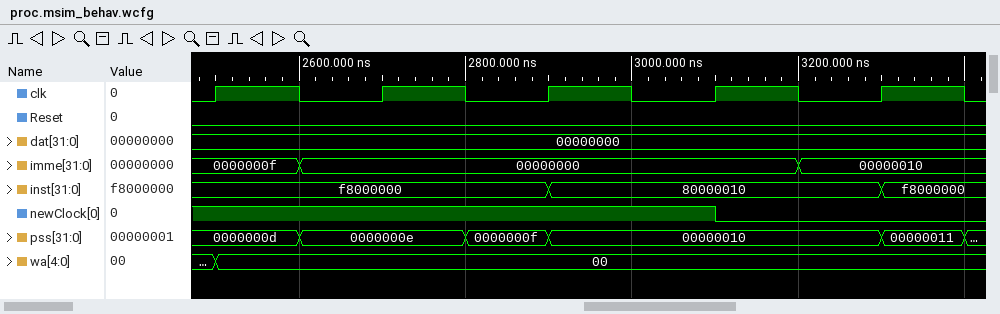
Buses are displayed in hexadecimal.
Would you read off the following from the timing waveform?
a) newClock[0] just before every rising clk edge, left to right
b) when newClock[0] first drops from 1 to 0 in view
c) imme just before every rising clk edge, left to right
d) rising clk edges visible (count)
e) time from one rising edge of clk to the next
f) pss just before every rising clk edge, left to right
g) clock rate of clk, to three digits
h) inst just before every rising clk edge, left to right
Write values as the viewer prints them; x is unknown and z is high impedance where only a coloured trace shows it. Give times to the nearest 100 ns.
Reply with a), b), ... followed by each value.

a) 1 1 1 1 0
b) 3100 ns
c) 0000000f, 00000000, 00000000, 00000000, 00000010
d) 5
e) 200 ns
f) 0000000d, 0000000e, 0000000f, 00000010, 00000010
g) 5.00 MHz
h) f8000000, f8000000, f8000000, 80000010, 80000010
